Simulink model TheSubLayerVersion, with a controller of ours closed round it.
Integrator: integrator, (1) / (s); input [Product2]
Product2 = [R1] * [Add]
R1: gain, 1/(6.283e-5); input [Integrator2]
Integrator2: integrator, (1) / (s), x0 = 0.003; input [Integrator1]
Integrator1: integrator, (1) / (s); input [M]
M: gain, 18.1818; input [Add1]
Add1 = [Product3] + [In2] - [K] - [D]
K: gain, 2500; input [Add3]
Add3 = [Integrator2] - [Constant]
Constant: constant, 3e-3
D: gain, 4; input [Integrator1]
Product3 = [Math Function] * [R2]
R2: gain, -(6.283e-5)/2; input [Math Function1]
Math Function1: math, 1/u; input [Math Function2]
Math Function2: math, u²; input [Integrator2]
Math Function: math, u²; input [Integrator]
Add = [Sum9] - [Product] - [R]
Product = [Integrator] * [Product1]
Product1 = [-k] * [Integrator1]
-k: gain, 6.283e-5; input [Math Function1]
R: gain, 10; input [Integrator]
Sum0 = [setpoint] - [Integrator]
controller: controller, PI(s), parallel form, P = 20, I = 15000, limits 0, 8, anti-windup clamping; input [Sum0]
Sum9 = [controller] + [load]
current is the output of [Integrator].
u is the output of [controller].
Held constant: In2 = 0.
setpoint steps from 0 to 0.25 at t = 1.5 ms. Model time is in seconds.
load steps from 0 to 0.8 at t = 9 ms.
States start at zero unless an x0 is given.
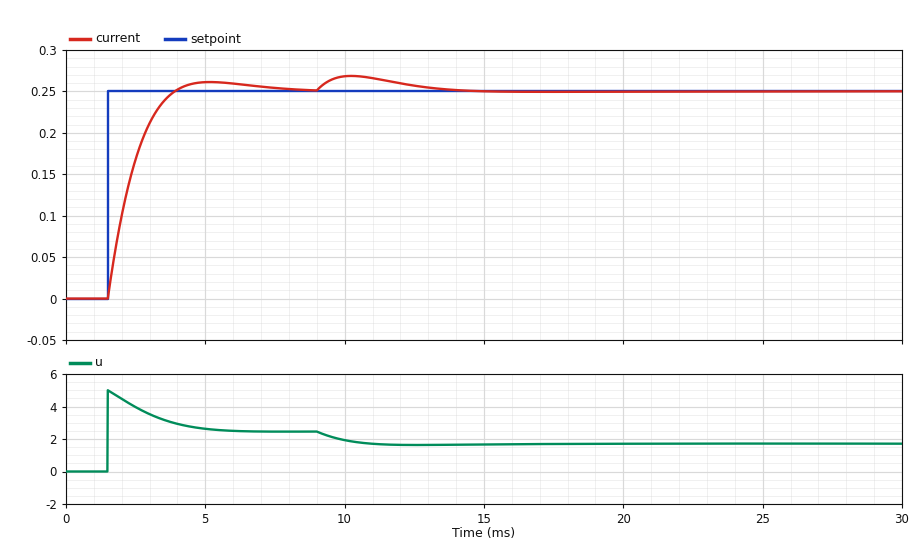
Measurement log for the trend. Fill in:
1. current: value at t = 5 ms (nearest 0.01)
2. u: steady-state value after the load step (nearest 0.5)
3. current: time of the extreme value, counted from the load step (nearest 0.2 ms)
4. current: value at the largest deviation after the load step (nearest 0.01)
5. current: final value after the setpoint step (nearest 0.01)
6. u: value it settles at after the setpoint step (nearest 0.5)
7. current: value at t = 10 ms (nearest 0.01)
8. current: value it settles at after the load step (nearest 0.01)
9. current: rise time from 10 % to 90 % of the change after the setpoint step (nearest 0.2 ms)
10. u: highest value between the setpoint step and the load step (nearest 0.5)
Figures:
0.26
1.5
1.2 ms
0.27
0.25
2.5
0.27
0.25
1.6 ms
5.0
